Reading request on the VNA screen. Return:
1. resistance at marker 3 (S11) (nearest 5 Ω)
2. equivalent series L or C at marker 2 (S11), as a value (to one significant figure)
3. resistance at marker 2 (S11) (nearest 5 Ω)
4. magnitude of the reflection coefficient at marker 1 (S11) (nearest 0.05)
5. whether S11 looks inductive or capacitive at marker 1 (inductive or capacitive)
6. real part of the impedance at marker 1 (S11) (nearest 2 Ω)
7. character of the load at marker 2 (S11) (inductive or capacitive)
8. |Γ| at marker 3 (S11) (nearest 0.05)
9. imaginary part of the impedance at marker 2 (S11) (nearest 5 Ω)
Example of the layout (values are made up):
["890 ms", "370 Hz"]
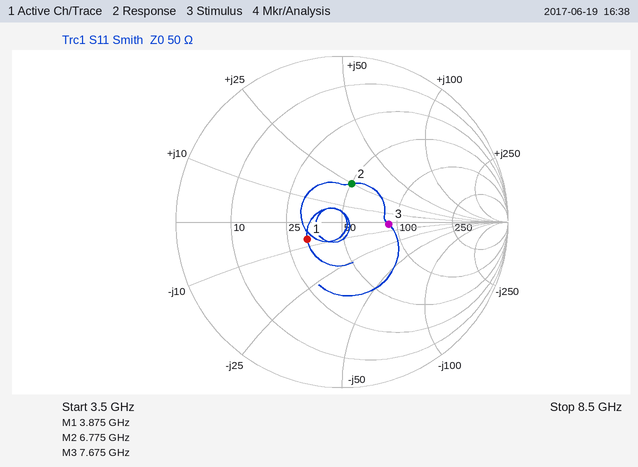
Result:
["90 Ω", "600 pH", "50 Ω", "0.25", "capacitive", "32 Ω", "inductive", "0.30", "+25 Ω"]
